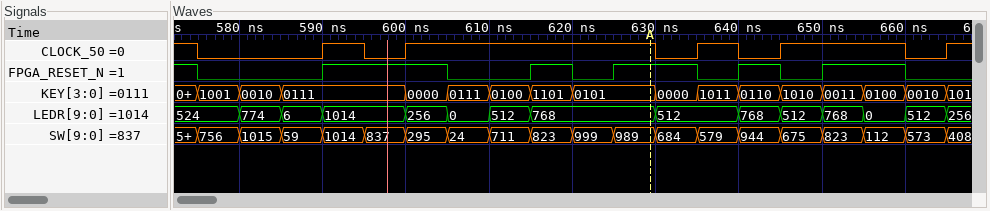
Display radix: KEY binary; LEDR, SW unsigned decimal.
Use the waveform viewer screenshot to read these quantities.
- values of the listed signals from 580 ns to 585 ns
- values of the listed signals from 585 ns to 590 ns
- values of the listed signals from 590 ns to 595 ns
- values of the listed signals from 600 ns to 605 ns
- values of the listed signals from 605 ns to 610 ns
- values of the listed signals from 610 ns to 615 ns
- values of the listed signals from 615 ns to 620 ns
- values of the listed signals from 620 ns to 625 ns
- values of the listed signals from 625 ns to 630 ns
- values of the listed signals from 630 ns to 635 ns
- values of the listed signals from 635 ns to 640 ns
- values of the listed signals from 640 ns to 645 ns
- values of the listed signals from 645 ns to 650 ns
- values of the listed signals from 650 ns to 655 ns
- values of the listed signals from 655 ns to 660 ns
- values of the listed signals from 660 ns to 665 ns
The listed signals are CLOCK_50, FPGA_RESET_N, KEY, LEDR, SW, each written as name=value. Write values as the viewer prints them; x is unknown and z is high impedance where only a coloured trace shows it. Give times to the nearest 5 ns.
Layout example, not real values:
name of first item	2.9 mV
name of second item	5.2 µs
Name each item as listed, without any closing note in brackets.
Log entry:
values of the listed signals from 580 ns to 585 ns	CLOCK_50=0, FPGA_RESET_N=0, KEY=0010, LEDR=774, SW=1015
values of the listed signals from 585 ns to 590 ns	CLOCK_50=0, FPGA_RESET_N=0, KEY=0111, LEDR=6, SW=59
values of the listed signals from 590 ns to 595 ns	CLOCK_50=1, FPGA_RESET_N=1, KEY=0111, LEDR=1014, SW=1014
values of the listed signals from 600 ns to 605 ns	CLOCK_50=1, FPGA_RESET_N=1, KEY=0000, LEDR=256, SW=295
values of the listed signals from 605 ns to 610 ns	CLOCK_50=1, FPGA_RESET_N=0, KEY=0111, LEDR=0, SW=24
values of the listed signals from 610 ns to 615 ns	CLOCK_50=1, FPGA_RESET_N=0, KEY=0100, LEDR=512, SW=711
values of the listed signals from 615 ns to 620 ns	CLOCK_50=1, FPGA_RESET_N=1, KEY=1101, LEDR=768, SW=823
values of the listed signals from 620 ns to 625 ns	CLOCK_50=1, FPGA_RESET_N=0, KEY=0101, LEDR=768, SW=999
values of the listed signals from 625 ns to 630 ns	CLOCK_50=1, FPGA_RESET_N=1, KEY=0101, LEDR=768, SW=989
values of the listed signals from 630 ns to 635 ns	CLOCK_50=0, FPGA_RESET_N=1, KEY=0000, LEDR=512, SW=684
values of the listed signals from 635 ns to 640 ns	CLOCK_50=1, FPGA_RESET_N=0, KEY=1011, LEDR=512, SW=579
values of the listed signals from 640 ns to 645 ns	CLOCK_50=0, FPGA_RESET_N=1, KEY=0110, LEDR=768, SW=944
values of the listed signals from 645 ns to 650 ns	CLOCK_50=1, FPGA_RESET_N=0, KEY=1010, LEDR=512, SW=675
values of the listed signals from 650 ns to 655 ns	CLOCK_50=1, FPGA_RESET_N=1, KEY=0011, LEDR=768, SW=823
values of the listed signals from 655 ns to 660 ns	CLOCK_50=1, FPGA_RESET_N=1, KEY=0100, LEDR=0, SW=112
values of the listed signals from 660 ns to 665 ns	CLOCK_50=0, FPGA_RESET_N=0, KEY=0010, LEDR=512, SW=573
